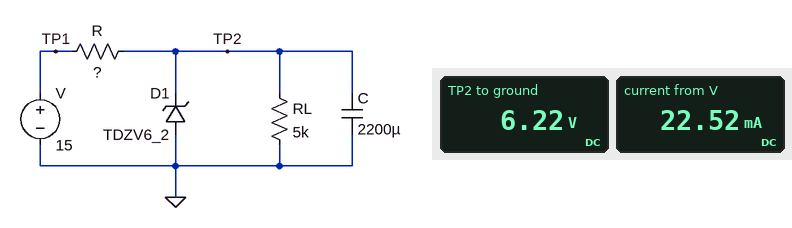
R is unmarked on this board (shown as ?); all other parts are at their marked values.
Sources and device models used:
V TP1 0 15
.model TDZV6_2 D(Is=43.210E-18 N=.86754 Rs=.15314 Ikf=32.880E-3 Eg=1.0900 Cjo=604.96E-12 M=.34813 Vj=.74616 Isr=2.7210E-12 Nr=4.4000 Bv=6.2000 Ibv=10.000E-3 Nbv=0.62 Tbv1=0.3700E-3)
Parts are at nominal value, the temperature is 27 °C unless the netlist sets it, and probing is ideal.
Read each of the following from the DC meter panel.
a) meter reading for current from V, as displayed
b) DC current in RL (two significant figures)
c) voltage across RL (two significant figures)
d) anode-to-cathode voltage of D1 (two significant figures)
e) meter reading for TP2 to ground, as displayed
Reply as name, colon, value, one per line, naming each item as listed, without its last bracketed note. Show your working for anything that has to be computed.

meter reading for current from V, as displayed: 22.52 mA
DC current in RL: (6.22 V) / 5 kΩ = 1.2 mA
voltage across RL: 6.22 V = 6.2 V
anode-to-cathode voltage of D1: 0 V - 6.22 V = -6.2 V
meter reading for TP2 to ground, as displayed: 6.22 V
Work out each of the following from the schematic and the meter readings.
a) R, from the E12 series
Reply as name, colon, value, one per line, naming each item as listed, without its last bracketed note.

R, from the E12 series: 390 Ω
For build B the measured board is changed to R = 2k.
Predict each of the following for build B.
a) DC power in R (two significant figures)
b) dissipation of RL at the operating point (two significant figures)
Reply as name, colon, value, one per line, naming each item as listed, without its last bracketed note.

DC power in R: 39 mW
dissipation of RL at the operating point: 7.6 mW
